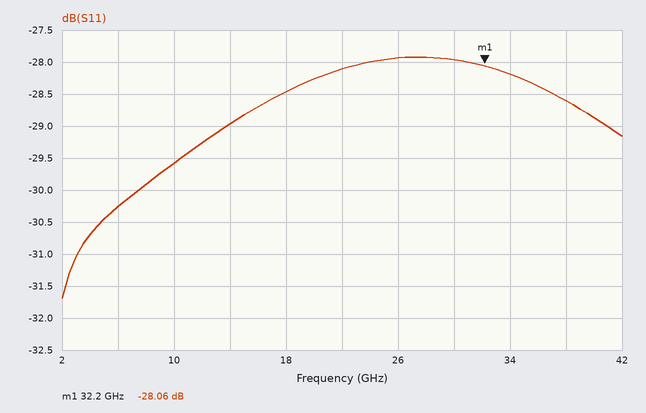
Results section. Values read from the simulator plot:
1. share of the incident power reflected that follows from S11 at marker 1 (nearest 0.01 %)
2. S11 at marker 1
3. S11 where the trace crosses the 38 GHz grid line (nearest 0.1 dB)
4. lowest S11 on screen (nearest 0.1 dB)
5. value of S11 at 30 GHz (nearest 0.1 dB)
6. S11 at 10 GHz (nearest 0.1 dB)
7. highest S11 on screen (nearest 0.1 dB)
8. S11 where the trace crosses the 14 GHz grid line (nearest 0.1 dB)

0.16 %
-28.06 dB
-28.6 dB
-31.7 dB
-28.0 dB
-29.6 dB
-27.9 dB
-29.0 dB
